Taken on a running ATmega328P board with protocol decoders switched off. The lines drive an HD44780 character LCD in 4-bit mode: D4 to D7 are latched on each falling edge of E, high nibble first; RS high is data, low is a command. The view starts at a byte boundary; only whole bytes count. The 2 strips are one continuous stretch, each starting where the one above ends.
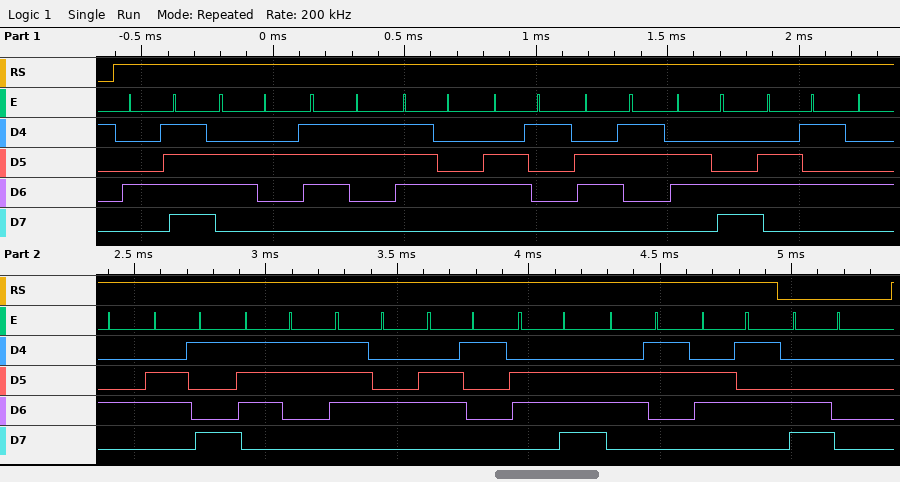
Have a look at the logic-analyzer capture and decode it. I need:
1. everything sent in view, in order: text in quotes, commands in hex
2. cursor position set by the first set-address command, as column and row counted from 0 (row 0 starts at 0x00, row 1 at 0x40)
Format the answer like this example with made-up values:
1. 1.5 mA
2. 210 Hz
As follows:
1. "ObstacleDistance" 0xC0
2. column 0, row 1
